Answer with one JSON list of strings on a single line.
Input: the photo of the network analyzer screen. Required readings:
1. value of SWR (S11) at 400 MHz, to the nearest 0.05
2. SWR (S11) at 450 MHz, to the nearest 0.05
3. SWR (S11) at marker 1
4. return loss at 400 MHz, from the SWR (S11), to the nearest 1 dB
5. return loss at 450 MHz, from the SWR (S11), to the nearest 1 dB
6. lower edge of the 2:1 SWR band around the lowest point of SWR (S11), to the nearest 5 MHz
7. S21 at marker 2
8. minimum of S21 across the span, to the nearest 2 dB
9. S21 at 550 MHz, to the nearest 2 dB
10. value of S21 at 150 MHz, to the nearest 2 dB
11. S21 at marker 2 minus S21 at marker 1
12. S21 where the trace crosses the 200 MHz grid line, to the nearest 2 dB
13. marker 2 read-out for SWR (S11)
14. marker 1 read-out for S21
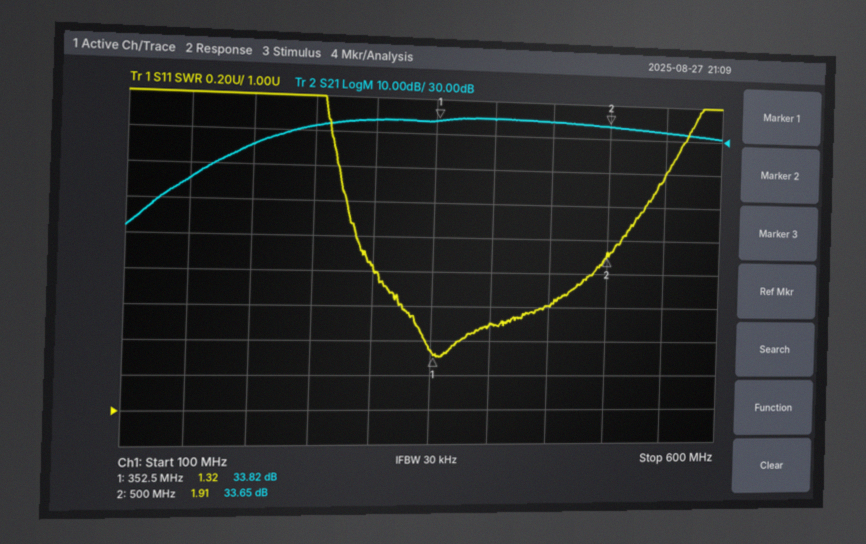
["1.50", "1.60", "1.32", "14 dB", "13 dB", "285 MHz", "33.65 dB", "2 dB", "32 dB", "16 dB", "-0.17 dB", "26 dB", "1.91", "33.82 dB"]
